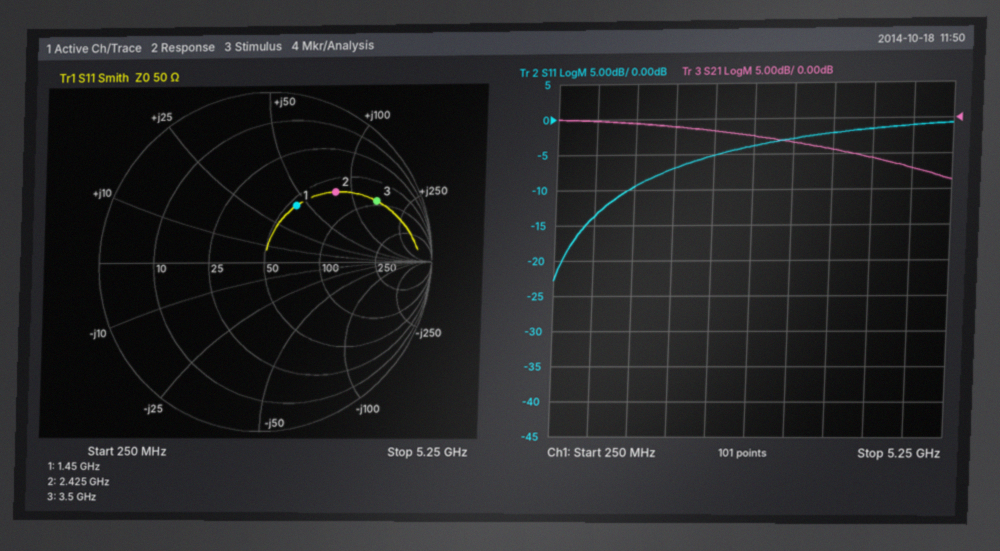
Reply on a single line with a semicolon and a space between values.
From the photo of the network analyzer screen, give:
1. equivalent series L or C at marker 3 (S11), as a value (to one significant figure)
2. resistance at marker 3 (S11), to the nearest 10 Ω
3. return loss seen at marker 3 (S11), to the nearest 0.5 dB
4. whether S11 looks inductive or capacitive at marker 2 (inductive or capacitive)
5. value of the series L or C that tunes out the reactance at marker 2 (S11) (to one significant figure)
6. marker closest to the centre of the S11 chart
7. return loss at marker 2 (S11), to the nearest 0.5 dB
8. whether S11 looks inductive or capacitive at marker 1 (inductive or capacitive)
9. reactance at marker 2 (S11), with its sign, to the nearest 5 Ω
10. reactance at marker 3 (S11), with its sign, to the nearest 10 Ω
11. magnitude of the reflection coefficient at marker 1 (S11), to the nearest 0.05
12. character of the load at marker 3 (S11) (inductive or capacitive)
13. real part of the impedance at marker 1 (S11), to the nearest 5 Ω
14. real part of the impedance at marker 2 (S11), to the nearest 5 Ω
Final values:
7 nH; 90 Ω; 2.5 dB; inductive; 800 fF; marker 1; 4.5 dB; inductive; +80 Ω; +150 Ω; 0.40; inductive; 55 Ω; 65 Ω
